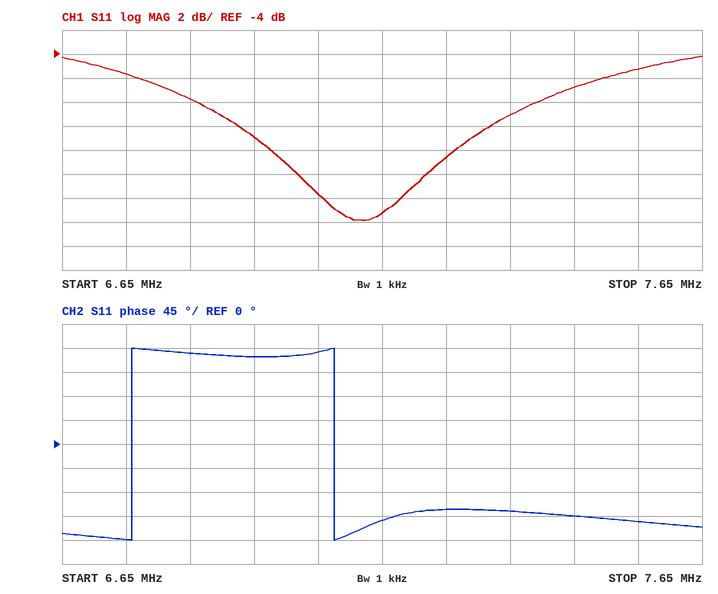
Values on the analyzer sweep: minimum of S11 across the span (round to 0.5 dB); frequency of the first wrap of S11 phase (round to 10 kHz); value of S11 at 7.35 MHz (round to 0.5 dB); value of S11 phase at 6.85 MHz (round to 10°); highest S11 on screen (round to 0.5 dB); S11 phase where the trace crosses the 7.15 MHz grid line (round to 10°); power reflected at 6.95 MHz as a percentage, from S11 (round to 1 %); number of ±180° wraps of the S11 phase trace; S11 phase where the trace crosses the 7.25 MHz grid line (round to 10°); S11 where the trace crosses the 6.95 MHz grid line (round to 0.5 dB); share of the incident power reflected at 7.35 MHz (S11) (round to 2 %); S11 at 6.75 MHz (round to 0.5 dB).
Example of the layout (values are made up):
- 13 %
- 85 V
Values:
- -18.0 dB
- 6.76 MHz
- -9.0 dB
- 170°
- -4.0 dB
- -140°
- 8 %
- 2
- -120°
- -11.0 dB
- 12 %
- -5.5 dB
